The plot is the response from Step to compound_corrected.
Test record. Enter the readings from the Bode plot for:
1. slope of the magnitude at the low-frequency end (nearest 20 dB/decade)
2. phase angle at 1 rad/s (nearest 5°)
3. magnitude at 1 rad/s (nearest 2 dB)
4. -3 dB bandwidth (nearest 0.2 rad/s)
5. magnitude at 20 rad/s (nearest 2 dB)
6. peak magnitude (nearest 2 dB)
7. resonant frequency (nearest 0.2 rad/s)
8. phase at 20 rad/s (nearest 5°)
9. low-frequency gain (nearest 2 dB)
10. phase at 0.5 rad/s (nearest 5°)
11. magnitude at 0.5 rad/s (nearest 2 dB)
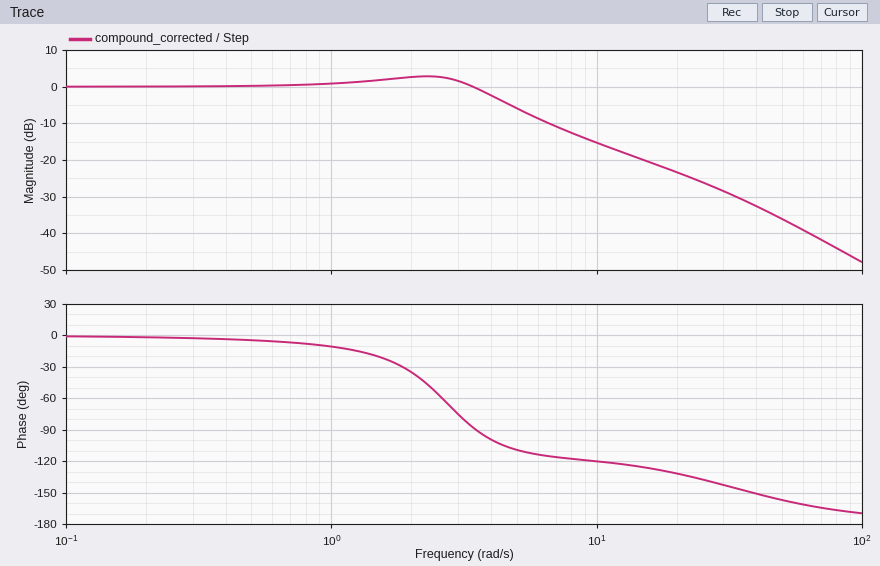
0 dB/decade
-10°
0 dB
4.2 rad/s
-24 dB
2 dB
2.2 rad/s
-130°
0 dB
-5°
0 dB
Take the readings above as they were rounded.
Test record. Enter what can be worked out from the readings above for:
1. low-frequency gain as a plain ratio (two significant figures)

1.0
